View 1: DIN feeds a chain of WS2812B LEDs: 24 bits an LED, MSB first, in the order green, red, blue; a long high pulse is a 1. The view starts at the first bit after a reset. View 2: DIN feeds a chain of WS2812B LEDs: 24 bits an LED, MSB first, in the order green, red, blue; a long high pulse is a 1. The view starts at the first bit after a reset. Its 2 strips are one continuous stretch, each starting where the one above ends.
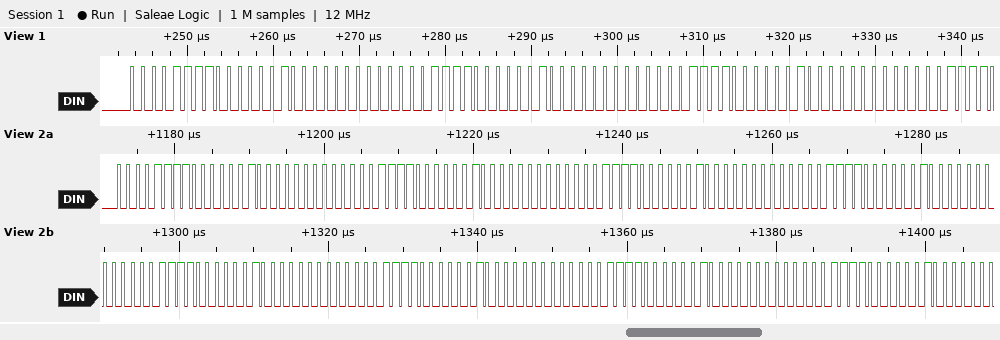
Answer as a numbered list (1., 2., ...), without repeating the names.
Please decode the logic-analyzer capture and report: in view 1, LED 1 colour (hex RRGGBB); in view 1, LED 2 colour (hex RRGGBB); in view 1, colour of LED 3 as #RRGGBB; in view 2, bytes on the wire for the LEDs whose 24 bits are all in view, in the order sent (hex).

1. #020F00
2. #020F00
3. #020F00
4. 0F 02 00 0F 02 00 0F 02 00 0F 02 00 0F 02 00 0F 02 00 0F 02 00
